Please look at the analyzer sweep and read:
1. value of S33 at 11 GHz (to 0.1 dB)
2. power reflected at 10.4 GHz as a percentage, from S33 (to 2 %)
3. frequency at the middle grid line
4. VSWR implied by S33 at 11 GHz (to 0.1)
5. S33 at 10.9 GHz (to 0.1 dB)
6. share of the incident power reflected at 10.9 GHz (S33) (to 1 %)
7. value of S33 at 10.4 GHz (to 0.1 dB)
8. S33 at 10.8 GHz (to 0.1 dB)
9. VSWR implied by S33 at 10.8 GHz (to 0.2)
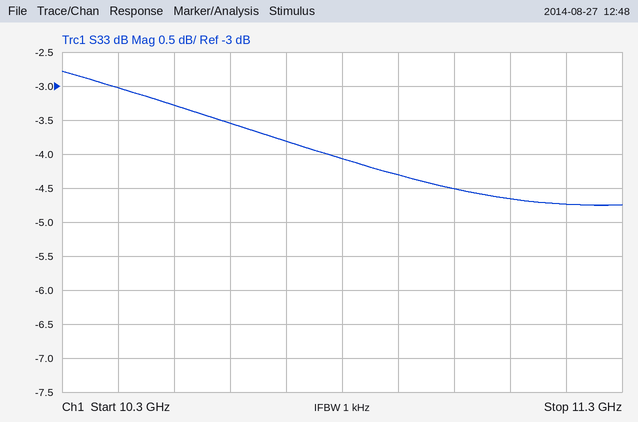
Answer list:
-4.5 dB
50 %
10.8 GHz
3.9
-4.3 dB
37 %
-3.0 dB
-4.1 dB
4.4
